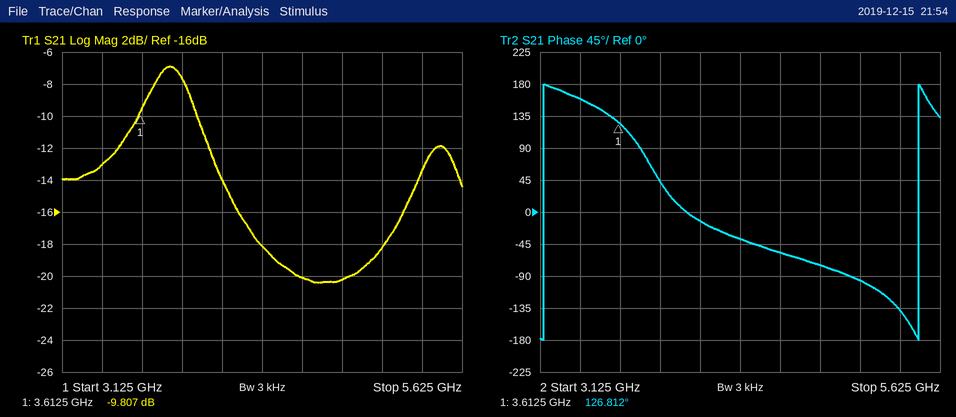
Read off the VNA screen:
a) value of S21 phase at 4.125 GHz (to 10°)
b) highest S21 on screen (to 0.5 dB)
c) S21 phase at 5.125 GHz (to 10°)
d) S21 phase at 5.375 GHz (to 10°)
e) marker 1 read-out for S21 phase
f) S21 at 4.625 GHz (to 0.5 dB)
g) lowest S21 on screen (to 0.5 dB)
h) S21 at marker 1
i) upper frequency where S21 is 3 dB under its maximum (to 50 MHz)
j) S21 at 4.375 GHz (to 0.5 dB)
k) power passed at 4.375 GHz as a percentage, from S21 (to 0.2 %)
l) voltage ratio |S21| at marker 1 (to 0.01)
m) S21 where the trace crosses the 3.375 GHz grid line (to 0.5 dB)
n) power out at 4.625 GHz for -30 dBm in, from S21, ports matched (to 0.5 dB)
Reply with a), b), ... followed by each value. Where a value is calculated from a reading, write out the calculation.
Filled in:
a) -10°
b) -7.0 dB
c) -100°
d) -140°
e) 126.812°
f) -20.0 dB
g) -20.5 dB
h) -9.807 dB
i) 3.95 GHz
j) -18.0 dB
k) 10^(-18/10) ≈ 1.6 %
l) 10^(-9.807/20) ≈ 0.32
m) -13.0 dB
n) -30 dBm + (-20.0 dB) = -50.0 dBm
